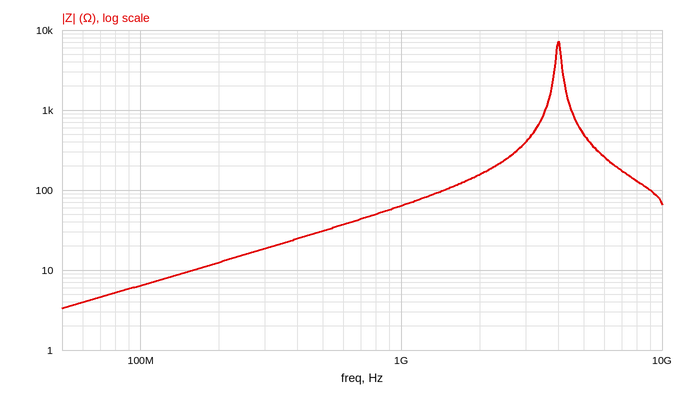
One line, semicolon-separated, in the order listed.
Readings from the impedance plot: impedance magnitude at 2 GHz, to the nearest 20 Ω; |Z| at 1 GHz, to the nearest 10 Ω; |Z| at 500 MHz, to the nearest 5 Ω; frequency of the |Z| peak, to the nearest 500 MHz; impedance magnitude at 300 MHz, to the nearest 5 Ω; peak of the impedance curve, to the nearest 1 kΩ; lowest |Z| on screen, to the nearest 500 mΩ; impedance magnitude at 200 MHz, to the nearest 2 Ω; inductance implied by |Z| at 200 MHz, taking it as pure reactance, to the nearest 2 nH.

160 Ω; 60 Ω; 30 Ω; 4.0 GHz; 20 Ω; 7 kΩ; 3.5 Ω; 12 Ω; 10 nH
